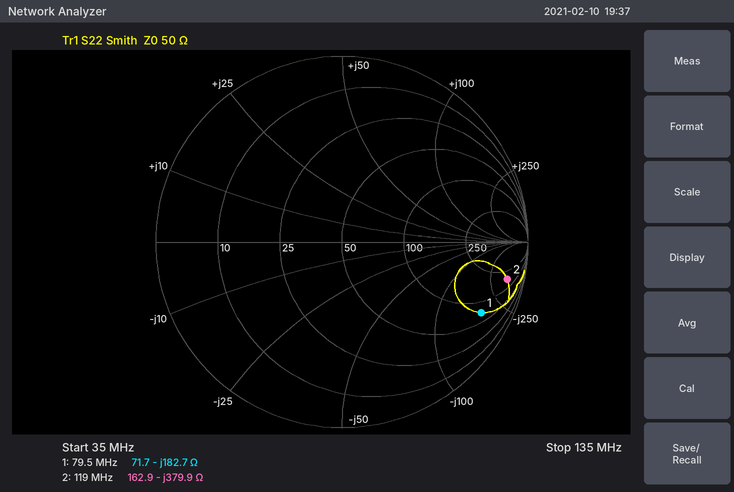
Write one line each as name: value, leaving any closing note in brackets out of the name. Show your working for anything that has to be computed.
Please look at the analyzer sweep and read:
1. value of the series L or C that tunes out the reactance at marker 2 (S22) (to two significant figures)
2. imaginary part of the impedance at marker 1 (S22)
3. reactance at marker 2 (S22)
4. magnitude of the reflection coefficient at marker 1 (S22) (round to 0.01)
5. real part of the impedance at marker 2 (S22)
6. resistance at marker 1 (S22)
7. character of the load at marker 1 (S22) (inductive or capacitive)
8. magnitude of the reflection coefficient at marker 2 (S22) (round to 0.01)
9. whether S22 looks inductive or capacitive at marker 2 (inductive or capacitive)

value of the series L or C that tunes out the reactance at marker 2 (S22): L = 379.9 Ω/(2π × 119 MHz) ≈ 508 nH, so 510 nH to two significant figures
imaginary part of the impedance at marker 1: -182.7 Ω
reactance at marker 2: -379.9 Ω
magnitude of the reflection coefficient at marker 1 (S22): 0.84
real part of the impedance at marker 2: 162.9 Ω
resistance at marker 1: 71.7 Ω
character of the load at marker 1 (S22): capacitive
magnitude of the reflection coefficient at marker 2 (S22): 0.91
whether S22 looks inductive or capacitive at marker 2: capacitive
